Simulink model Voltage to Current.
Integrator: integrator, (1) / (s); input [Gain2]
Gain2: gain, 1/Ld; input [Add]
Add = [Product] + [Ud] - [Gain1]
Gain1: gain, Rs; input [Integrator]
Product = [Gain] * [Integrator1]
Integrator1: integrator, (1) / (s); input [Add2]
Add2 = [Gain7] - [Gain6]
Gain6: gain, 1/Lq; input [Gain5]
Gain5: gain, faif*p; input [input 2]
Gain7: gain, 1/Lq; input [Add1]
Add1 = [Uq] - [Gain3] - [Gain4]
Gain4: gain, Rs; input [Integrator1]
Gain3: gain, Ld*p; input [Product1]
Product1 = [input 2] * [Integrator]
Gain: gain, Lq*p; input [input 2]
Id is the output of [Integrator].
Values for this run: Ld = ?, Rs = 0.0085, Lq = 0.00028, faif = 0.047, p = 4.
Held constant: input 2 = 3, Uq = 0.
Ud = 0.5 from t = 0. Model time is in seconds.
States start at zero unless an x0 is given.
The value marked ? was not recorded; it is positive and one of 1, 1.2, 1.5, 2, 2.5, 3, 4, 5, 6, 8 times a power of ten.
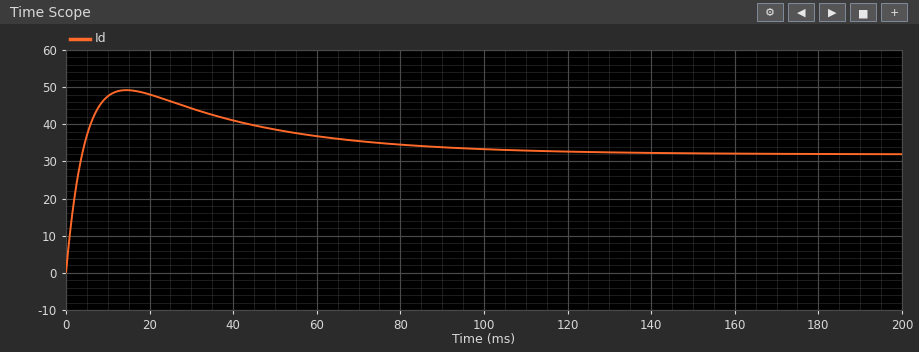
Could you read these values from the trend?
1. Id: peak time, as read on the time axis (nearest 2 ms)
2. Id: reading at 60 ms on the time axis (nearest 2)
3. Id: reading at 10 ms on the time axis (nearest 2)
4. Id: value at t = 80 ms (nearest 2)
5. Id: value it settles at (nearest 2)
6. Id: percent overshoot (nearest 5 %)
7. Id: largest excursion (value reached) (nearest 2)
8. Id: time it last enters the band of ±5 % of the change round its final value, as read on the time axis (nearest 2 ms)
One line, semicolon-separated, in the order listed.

14 ms; 36; 48; 34; 32; 55 %; 50; 96 ms
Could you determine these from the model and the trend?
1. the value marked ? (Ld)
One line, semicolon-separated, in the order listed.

4e-05
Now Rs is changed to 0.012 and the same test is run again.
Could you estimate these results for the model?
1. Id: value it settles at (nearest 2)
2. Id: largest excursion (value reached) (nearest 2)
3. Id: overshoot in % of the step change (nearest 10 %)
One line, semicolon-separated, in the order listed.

28; 36; 30 %
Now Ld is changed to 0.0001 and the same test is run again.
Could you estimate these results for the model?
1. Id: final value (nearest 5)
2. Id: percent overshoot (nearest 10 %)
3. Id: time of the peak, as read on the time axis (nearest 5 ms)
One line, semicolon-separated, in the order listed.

30; 40 %; 30 ms
